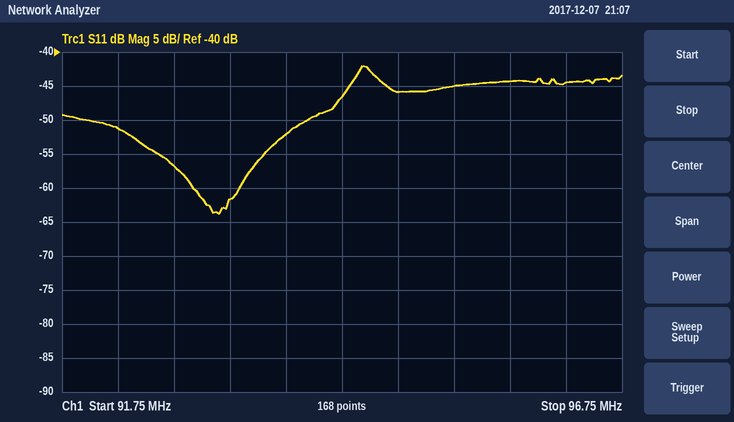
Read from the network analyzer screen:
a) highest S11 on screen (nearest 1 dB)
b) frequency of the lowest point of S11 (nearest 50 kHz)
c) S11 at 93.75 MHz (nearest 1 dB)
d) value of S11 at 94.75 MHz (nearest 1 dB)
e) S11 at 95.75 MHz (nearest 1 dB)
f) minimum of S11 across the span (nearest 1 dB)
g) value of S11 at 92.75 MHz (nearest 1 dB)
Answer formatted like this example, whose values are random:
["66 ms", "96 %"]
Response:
["-42 dB", "93.15 MHz", "-52 dB", "-46 dB", "-44 dB", "-64 dB", "-57 dB"]
